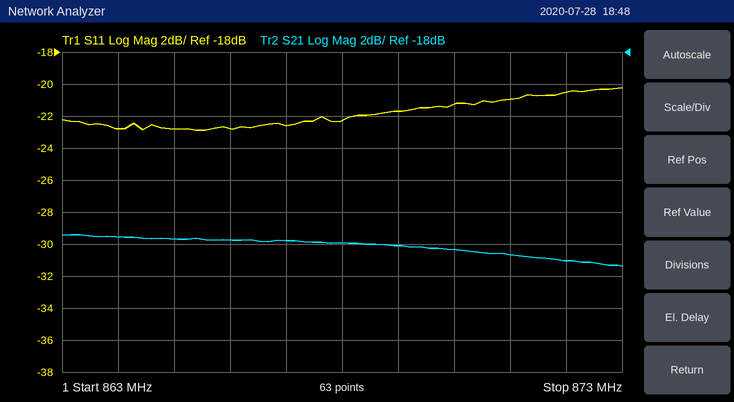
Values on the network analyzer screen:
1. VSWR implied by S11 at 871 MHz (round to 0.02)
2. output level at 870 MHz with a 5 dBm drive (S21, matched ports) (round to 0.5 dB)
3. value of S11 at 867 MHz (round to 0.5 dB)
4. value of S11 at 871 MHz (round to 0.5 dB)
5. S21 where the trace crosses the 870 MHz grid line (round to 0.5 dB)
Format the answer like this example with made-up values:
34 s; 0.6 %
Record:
1.20; -25.5 dBm; -22.5 dB; -21.0 dB; -30.5 dB
